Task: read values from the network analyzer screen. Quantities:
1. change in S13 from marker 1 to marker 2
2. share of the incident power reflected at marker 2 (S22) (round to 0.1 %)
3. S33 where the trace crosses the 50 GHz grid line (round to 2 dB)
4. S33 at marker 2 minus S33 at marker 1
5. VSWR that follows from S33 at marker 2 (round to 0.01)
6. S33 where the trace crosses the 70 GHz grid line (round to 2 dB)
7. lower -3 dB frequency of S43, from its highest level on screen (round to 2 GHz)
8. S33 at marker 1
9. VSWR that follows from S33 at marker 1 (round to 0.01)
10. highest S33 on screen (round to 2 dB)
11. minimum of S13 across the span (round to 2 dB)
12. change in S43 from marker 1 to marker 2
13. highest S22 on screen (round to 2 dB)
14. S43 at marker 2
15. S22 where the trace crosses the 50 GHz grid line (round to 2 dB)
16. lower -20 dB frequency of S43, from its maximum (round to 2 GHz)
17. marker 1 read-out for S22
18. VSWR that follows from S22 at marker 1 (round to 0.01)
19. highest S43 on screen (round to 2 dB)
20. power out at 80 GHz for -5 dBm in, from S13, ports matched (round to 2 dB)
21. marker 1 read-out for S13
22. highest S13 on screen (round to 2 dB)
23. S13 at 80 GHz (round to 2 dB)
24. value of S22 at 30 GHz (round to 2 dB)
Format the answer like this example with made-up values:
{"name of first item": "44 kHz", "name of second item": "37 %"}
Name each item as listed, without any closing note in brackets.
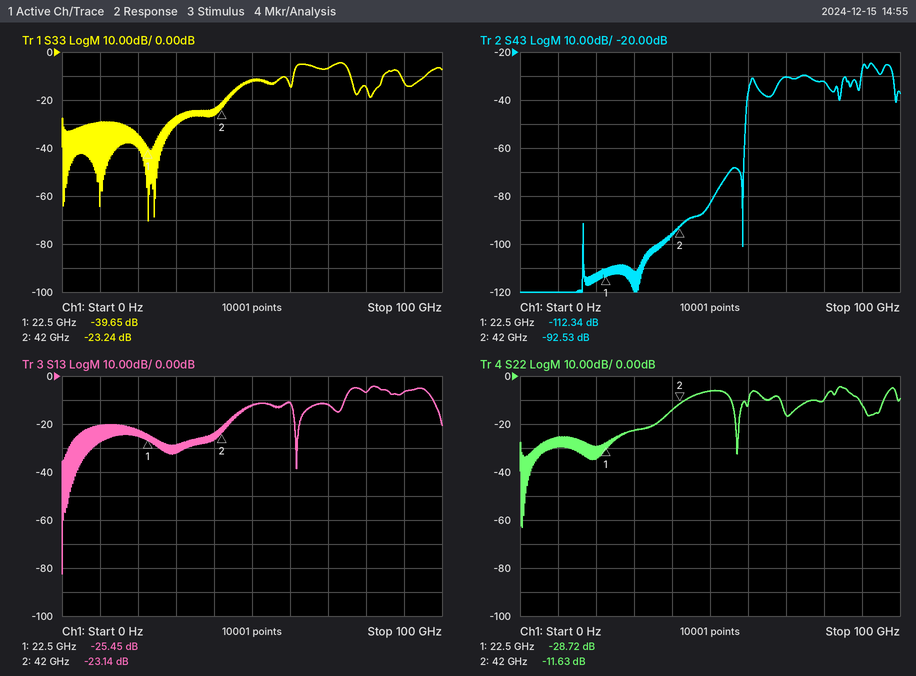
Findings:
{"change in S13 from marker 1 to marker 2": "2.31 dB", "share of the incident power reflected at marker 2 (S22)": "6.9 %", "S33 where the trace crosses the 50 GHz grid line": "-12 dB", "S33 at marker 2 minus S33 at marker 1": "16.41 dB", "VSWR that follows from S33 at marker 2": "1.15", "S33 where the trace crosses the 70 GHz grid line": "-6 dB", "lower -3 dB frequency of S43, from its highest level on screen": "90 GHz", "S33 at marker 1": "-39.65 dB", "VSWR that follows from S33 at marker 1": "1.02", "highest S33 on screen": "-4 dB", "minimum of S13 across the span": "-82 dB", "change in S43 from marker 1 to marker 2": "19.81 dB", "highest S22 on screen": "-4 dB", "S43 at marker 2": "-92.53 dB", "S22 where the trace crosses the 50 GHz grid line": "-6 dB", "lower -20 dB frequency of S43, from its maximum": "60 GHz", "marker 1 read-out for S22": "-28.72 dB", "VSWR that follows from S22 at marker 1": "1.08", "highest S43 on screen": "-24 dB", "power out at 80 GHz for -5 dBm in, from S13, ports matched": "-12 dBm", "marker 1 read-out for S13": "-25.45 dB", "highest S13 on screen": "-4 dB", "S13 at 80 GHz": "-6 dB", "value of S22 at 30 GHz": "-22 dB"}
